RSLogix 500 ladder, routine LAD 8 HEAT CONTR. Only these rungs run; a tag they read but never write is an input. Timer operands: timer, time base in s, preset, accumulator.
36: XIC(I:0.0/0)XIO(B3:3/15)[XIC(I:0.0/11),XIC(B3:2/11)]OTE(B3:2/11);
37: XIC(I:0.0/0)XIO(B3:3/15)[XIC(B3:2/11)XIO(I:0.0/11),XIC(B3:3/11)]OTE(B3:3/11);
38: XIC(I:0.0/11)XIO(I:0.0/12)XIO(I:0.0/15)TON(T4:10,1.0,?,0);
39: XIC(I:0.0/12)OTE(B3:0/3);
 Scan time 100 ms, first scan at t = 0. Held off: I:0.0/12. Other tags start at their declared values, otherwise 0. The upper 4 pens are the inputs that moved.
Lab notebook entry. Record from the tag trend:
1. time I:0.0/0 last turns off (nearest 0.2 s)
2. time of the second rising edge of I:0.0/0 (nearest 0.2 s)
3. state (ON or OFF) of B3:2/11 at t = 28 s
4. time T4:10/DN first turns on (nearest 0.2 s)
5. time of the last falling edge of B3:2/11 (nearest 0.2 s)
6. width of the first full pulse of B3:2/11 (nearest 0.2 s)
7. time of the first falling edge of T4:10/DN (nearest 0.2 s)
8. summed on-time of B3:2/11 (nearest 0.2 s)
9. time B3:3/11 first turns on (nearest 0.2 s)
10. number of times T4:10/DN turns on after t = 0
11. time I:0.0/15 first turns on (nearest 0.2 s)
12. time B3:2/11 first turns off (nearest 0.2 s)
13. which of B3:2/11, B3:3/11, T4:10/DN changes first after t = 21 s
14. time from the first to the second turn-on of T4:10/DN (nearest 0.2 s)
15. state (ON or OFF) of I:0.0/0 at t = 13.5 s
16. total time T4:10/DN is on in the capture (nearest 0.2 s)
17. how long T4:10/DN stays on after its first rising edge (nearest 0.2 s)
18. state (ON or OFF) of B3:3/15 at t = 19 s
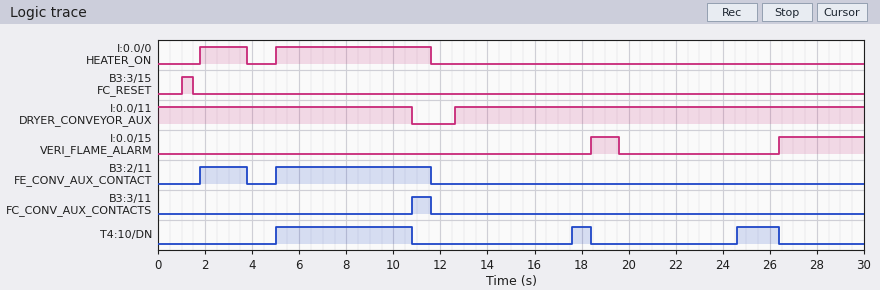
11.6 s
5.0 s
OFF
5.0 s
11.6 s
2.0 s
10.8 s
8.6 s
10.8 s
3
18.4 s
3.8 s
T4:10/DN
12.6 s
OFF
8.4 s
5.8 s
OFF
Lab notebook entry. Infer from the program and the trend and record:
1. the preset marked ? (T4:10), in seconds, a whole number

5 s
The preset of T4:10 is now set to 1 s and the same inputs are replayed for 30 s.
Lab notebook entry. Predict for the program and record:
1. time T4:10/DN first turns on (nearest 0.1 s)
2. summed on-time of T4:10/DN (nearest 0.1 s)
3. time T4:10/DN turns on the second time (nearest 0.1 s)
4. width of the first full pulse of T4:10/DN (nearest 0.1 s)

1.0 s
20.4 s
13.6 s
9.8 s
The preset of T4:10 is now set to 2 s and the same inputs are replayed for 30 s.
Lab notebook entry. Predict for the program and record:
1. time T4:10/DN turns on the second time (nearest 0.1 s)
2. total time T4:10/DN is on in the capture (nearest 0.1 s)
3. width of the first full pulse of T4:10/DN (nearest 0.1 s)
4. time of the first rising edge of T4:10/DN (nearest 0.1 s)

14.6 s
17.4 s
8.8 s
2.0 s
